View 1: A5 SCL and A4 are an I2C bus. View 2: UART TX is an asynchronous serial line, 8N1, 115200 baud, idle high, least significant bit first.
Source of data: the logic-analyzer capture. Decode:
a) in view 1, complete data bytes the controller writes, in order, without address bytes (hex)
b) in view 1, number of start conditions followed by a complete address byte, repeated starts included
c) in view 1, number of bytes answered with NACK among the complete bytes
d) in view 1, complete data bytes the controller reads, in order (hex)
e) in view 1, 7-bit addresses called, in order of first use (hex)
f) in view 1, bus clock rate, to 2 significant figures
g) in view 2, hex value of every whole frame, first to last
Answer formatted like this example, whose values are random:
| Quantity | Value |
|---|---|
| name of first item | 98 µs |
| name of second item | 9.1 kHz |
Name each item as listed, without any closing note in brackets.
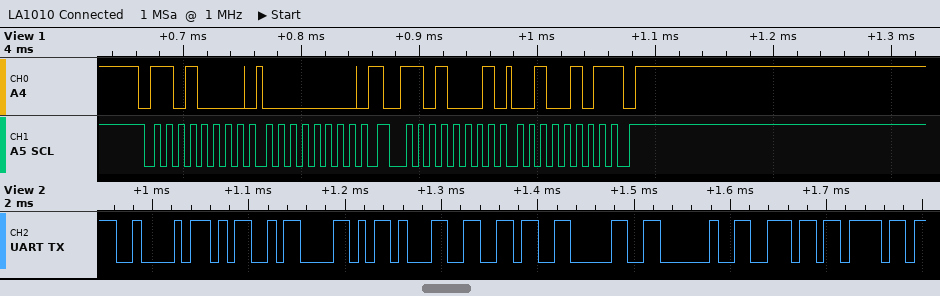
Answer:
| Quantity | Value |
|---|---|
| in view 1, complete data bytes the controller writes, in order, without address bytes | 00 |
| in view 1, number of start conditions followed by a complete address byte, repeated starts included | 2 |
| in view 1, number of bytes answered with NACK among the complete bytes | 1 |
| in view 1, complete data bytes the controller reads, in order | 25 |
| in view 1, 7-bit addresses called, in order of first use | 0x68 |
| in view 1, bus clock rate, to 2 significant figures | 100 kHz |
| in view 2, hex value of every whole frame, first to last | 0x42 0x4D 0x58 0x31 0x36 0x30 0x20 0x6E 0x6F |
